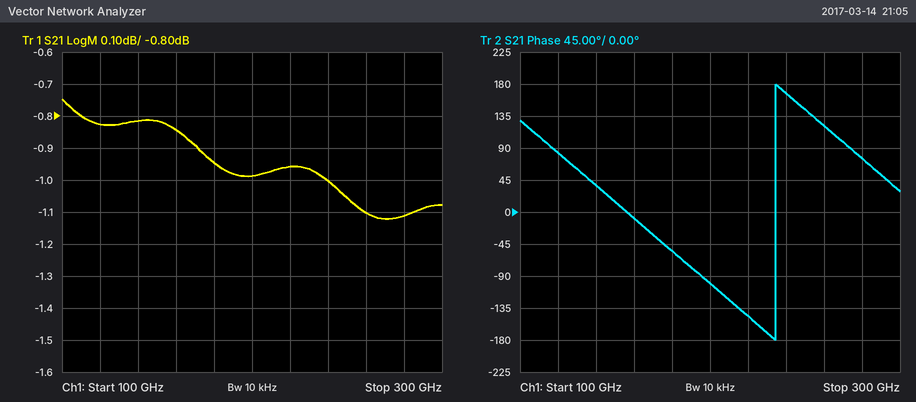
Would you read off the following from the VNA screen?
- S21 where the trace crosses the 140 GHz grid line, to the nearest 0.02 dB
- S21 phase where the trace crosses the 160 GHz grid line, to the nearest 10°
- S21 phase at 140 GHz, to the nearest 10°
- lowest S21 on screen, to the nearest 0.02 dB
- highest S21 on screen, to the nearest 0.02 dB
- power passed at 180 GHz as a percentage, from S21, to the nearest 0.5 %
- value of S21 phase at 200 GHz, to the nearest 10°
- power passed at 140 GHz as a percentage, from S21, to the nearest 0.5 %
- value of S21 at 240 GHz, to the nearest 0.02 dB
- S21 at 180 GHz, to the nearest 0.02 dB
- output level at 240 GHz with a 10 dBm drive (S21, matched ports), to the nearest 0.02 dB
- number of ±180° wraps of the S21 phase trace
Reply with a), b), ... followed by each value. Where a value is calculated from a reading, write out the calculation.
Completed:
a) -0.82 dB
b) -10°
c) 40°
d) -1.12 dB
e) -0.74 dB
f) 10^(-0.94/10) ≈ 80.5 %
g) -100°
h) 10^(-0.82/10) ≈ 82.8 %, so 83.0 % to the nearest 0.5 %
i) -1.00 dB
j) -0.94 dB
k) 10 dBm + (-1.00 dB) = 9.00 dBm
l) 1
